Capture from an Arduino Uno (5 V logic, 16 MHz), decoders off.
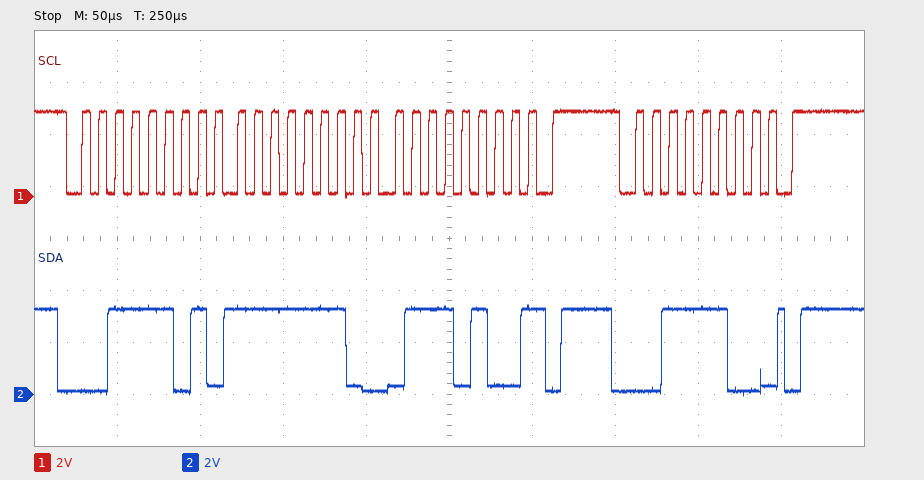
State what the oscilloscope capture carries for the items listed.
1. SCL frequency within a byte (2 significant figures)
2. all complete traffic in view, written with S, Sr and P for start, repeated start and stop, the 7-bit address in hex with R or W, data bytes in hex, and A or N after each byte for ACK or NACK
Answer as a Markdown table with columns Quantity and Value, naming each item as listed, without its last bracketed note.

| Quantity | Value |
|---|---|
| SCL frequency within a byte | 100 kHz |
| all complete traffic in view, written with S, Sr and P for start, repeated start and stop, the 7-bit address in hex with R or W, data bytes in hex, and A or N after each byte for ACK or NACK | S 1ER A FE A 74 N P S 1EW A P |
